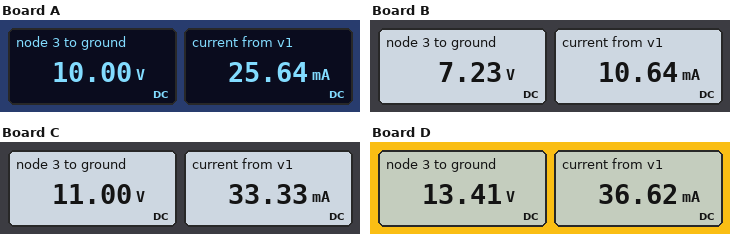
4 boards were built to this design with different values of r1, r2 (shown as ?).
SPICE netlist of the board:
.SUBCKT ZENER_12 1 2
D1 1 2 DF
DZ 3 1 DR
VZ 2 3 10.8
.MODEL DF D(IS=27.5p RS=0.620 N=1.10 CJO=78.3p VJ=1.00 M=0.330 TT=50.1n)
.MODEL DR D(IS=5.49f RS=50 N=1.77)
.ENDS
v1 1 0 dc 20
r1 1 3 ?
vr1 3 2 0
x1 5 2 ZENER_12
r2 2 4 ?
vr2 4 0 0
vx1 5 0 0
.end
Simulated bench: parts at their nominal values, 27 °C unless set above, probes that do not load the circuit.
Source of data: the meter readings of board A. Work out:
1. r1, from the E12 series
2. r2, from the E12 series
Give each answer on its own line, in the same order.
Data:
390 Ω
390 Ω
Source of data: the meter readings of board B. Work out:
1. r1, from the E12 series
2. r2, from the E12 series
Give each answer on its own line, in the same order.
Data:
1.2 kΩ
680 Ω
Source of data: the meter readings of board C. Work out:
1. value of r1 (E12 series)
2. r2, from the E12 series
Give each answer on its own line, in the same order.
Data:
270 Ω
330 Ω
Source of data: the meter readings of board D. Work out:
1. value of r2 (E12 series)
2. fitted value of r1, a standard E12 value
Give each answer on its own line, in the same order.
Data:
1.2 kΩ
180 Ω
